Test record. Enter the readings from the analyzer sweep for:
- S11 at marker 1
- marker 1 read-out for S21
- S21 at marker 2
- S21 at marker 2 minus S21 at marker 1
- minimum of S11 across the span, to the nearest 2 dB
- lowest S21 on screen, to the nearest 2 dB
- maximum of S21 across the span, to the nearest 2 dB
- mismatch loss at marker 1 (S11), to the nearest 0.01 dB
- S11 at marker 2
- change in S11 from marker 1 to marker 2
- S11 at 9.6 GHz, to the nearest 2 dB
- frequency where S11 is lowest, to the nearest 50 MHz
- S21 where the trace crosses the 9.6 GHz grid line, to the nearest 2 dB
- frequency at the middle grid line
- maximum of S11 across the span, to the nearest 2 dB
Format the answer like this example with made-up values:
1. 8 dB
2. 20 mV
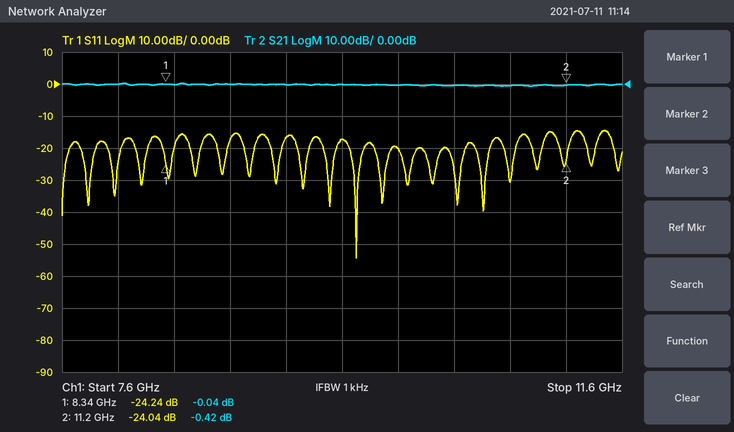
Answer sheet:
1. -24.24 dB
2. -0.04 dB
3. -0.42 dB
4. -0.38 dB
5. -54 dB
6. 0 dB
7. 0 dB
8. 0.02 dB
9. -24.04 dB
10. 0.20 dB
11. -18 dB
12. 9.70 GHz
13. 0 dB
14. 9.6 GHz
15. -14 dB
